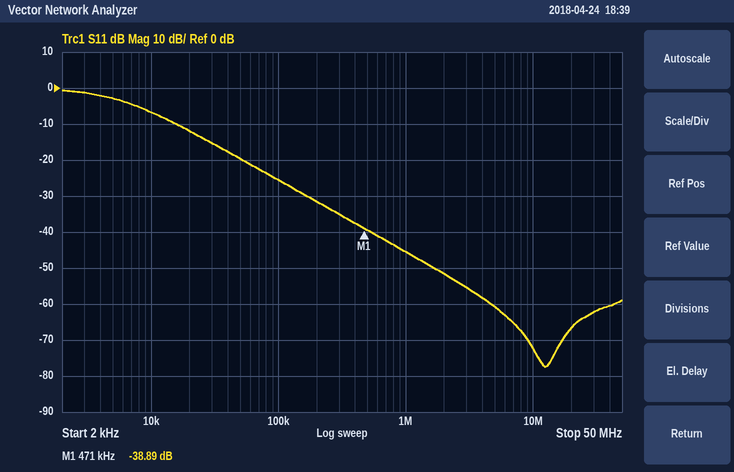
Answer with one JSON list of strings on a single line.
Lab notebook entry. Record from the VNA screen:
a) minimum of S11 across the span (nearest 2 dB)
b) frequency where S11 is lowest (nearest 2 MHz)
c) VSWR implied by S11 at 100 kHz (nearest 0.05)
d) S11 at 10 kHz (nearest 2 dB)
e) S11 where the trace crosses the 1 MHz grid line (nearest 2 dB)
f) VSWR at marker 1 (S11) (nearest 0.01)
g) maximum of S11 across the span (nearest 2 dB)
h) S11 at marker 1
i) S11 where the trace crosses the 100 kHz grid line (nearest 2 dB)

["-78 dB", "12 MHz", "1.10", "-6 dB", "-46 dB", "1.02", "0 dB", "-38.89 dB", "-26 dB"]
